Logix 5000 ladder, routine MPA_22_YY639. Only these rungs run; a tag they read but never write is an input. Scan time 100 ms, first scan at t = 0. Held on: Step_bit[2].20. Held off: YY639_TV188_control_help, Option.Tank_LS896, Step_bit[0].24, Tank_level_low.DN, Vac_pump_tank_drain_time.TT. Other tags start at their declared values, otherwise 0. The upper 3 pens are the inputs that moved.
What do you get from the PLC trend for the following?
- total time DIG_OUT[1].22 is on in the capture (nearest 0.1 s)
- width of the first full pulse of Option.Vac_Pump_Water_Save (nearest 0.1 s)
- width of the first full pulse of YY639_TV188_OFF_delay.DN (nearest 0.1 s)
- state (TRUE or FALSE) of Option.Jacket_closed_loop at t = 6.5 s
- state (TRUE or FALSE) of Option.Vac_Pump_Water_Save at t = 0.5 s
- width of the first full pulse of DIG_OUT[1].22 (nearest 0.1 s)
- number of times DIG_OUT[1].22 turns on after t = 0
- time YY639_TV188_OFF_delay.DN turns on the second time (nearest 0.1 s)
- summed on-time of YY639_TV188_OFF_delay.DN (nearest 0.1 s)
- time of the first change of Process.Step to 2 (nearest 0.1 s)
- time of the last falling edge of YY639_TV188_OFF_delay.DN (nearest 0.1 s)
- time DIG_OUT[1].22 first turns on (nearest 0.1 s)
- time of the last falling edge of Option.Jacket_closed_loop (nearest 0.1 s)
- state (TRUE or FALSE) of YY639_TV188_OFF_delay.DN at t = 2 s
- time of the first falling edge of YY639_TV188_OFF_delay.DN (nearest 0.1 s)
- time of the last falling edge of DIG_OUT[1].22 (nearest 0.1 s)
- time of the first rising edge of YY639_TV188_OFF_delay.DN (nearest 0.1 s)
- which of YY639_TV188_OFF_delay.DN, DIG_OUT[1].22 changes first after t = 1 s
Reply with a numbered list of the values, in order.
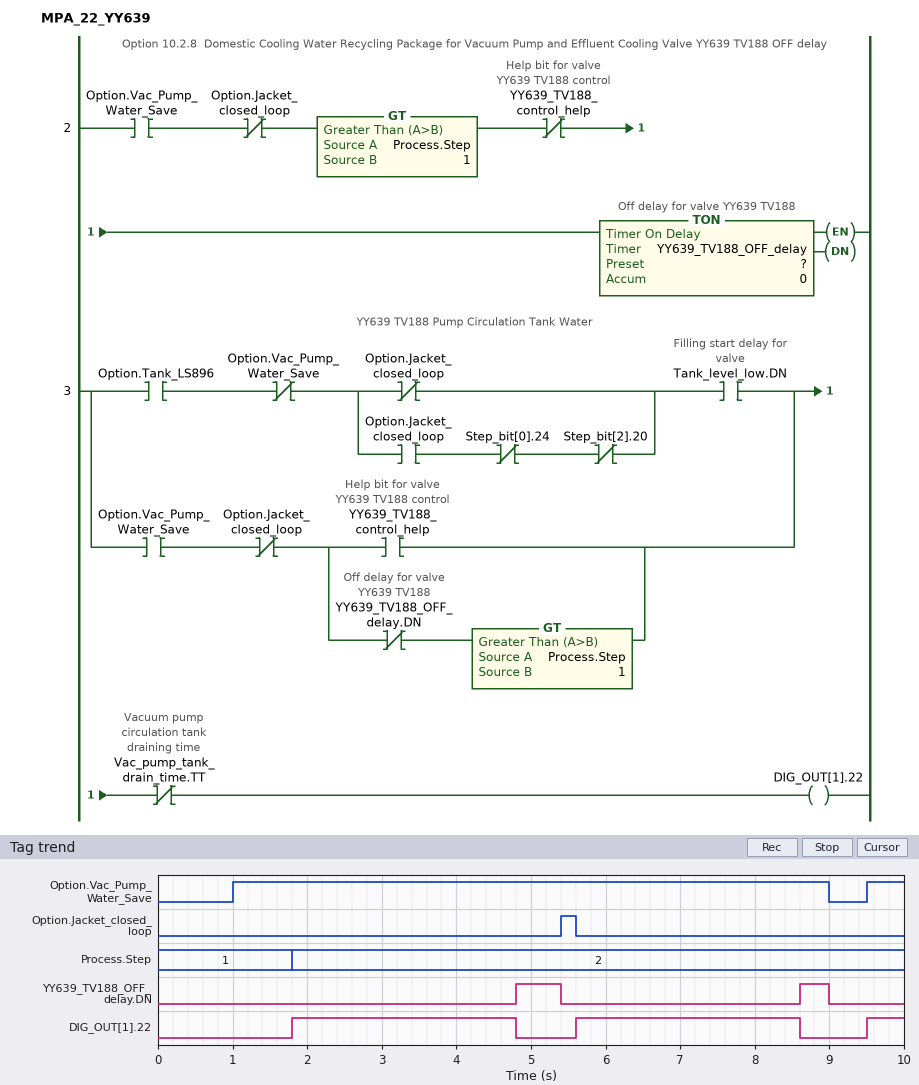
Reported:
1. 6.5 s
2. 8.0 s
3. 0.6 s
4. FALSE
5. FALSE
6. 3.0 s
7. 3
8. 8.6 s
9. 1.0 s
10. 1.8 s
11. 9.0 s
12. 1.8 s
13. 5.6 s
14. FALSE
15. 5.4 s
16. 8.6 s
17. 4.8 s
18. DIG_OUT[1].22
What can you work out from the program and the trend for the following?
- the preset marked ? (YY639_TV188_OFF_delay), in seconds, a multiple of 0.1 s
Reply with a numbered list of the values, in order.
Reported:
1. 3.0 s
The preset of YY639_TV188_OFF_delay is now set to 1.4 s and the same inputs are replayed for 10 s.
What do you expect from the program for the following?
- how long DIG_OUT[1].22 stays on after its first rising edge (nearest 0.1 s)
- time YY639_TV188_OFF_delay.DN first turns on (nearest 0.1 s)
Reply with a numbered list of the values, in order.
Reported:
1. 1.4 s
2. 3.2 s
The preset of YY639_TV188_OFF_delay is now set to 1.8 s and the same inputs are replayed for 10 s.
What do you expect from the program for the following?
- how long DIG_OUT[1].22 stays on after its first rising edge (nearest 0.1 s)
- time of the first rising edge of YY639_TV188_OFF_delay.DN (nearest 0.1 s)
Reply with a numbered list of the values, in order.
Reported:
1. 1.8 s
2. 3.6 s
